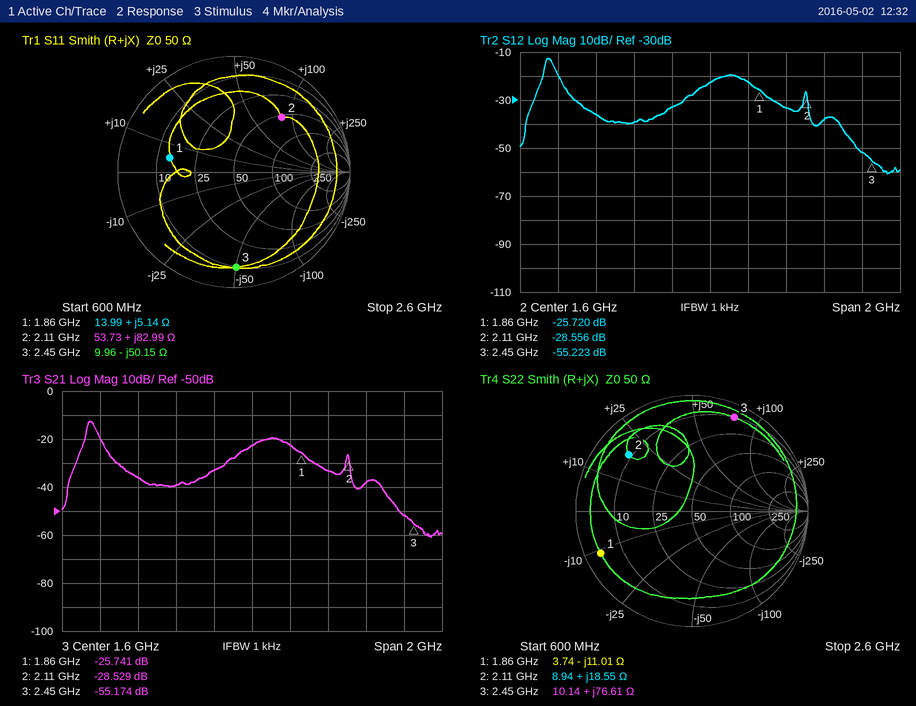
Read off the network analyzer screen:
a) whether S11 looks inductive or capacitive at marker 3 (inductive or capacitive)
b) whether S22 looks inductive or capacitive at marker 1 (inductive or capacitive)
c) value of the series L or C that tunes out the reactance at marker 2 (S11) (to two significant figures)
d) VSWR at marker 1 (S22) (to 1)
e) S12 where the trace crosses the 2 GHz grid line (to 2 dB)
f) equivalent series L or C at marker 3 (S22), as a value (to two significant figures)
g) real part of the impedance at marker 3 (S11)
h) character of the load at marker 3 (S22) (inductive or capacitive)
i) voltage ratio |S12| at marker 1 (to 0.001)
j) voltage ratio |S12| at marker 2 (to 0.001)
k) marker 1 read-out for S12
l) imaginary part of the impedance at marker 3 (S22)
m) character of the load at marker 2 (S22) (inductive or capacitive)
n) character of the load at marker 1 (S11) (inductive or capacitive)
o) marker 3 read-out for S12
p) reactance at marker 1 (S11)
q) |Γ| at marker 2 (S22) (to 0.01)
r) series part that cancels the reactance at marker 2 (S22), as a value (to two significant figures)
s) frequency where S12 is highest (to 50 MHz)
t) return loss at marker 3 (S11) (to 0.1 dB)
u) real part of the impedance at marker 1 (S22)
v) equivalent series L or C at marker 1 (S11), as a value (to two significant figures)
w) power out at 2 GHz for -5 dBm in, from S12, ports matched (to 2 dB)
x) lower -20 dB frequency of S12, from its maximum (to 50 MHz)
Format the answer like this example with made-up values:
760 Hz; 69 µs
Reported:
capacitive; capacitive; 910 fF; 14; -34 dB; 5.0 nH; 9.96 Ω; inductive; 0.052; 0.037; -25.720 dB; +76.61 Ω; inductive; inductive; -55.223 dB; +5.14 Ω; 0.73; 4.1 pF; 750 MHz; 1.7 dB; 3.74 Ω; 440 pH; -38 dBm; 650 MHz
